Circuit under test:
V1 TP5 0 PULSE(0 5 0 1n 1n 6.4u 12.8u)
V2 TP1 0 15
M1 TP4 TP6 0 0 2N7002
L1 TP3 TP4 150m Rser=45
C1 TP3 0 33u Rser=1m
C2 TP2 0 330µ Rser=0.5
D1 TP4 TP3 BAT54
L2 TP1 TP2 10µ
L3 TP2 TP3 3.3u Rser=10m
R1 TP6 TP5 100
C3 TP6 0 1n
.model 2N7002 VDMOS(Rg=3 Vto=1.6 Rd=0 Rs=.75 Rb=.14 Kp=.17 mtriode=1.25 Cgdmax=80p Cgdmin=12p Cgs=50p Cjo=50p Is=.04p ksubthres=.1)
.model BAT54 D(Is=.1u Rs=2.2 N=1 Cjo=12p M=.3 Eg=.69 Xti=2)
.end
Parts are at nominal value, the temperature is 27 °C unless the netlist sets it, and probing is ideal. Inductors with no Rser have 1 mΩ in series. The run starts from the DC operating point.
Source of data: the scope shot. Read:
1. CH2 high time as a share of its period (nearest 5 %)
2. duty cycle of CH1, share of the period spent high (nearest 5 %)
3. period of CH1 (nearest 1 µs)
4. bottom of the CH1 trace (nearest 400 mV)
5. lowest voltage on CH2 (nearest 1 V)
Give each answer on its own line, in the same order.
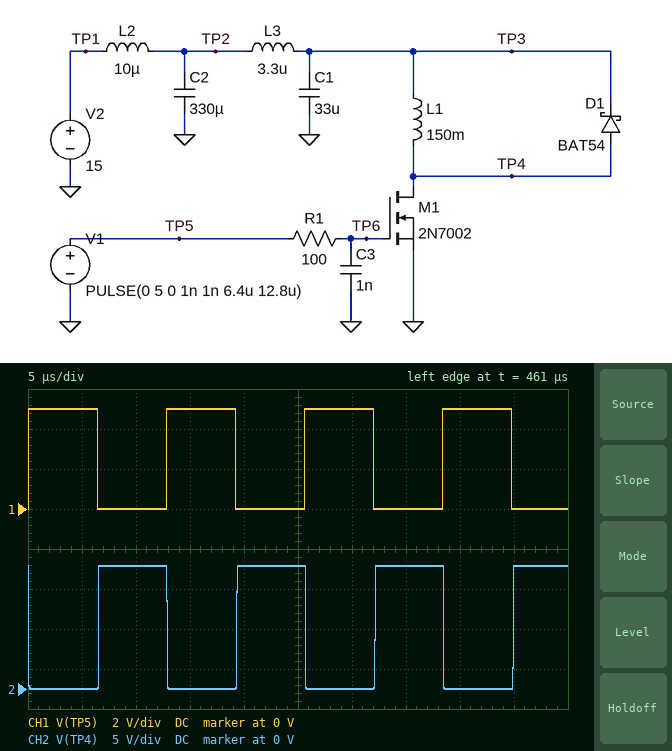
50 %
50 %
13 µs
0 V
0 V
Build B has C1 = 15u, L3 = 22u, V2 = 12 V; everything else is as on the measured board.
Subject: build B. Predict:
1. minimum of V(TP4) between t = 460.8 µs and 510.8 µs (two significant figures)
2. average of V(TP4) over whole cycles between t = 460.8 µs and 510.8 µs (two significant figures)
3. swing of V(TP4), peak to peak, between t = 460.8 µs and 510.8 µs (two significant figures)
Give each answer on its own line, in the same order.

29 mV
6.1 V
12 V
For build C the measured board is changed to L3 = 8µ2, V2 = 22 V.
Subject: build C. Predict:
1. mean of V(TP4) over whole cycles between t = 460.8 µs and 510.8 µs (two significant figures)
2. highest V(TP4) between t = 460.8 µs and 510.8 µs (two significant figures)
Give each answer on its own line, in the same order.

11 V
22 V
